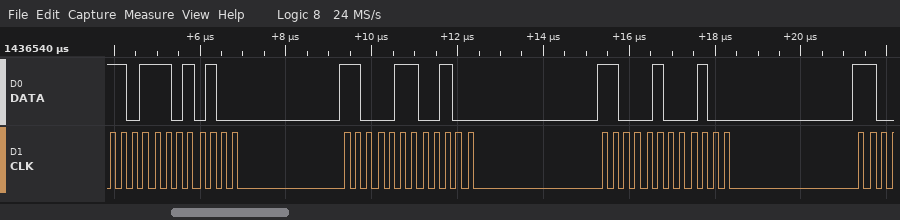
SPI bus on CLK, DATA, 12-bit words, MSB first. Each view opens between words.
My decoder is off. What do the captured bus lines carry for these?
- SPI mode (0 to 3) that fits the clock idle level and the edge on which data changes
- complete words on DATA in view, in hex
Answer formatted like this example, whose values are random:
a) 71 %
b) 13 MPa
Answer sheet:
a) 0
b) DD4, C64, C44
